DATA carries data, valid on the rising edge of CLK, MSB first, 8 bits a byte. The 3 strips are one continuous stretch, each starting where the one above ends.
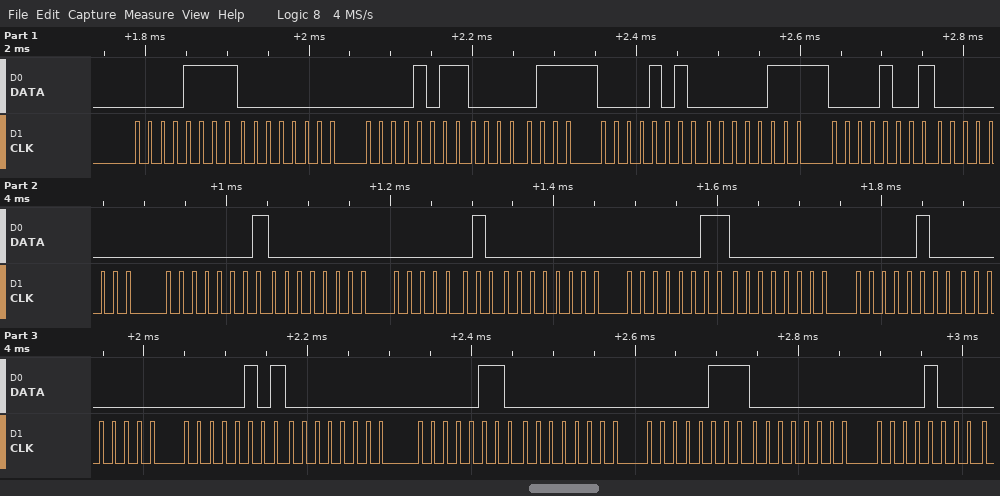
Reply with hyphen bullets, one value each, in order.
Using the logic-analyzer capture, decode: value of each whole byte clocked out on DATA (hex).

- 0F 00 0B 07 0A 07 09 00 01 00 02 00 03 00 04 00 05 00 06 00 07 00 08
